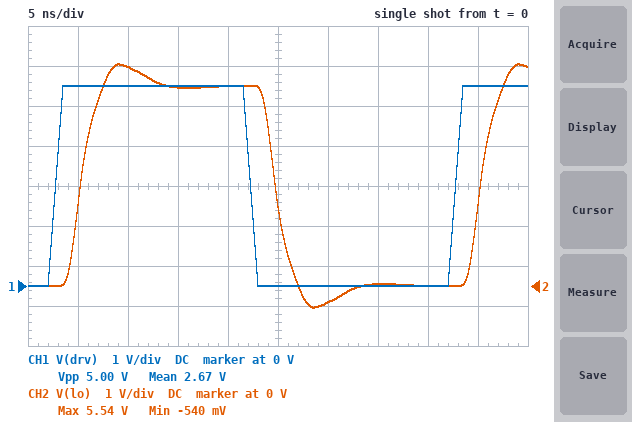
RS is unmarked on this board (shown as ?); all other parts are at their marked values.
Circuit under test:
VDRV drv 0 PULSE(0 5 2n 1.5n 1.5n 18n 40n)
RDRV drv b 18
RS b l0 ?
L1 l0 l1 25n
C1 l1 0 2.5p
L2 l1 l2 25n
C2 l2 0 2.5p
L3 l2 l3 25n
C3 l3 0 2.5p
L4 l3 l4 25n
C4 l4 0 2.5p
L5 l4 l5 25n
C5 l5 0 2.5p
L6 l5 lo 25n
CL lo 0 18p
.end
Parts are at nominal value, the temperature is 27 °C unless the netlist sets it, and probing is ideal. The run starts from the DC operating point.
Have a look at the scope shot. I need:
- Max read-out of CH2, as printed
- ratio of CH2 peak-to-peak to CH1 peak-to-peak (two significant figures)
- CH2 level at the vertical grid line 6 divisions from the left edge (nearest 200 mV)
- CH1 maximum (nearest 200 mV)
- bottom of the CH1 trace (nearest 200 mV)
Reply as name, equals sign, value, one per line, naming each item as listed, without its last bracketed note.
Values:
Max read-out of CH2, as printed = 5.54 V
ratio of CH2 peak-to-peak to CH1 peak-to-peak = 1.2
CH2 level at the vertical grid line 6 divisions from the left edge = -400 mV
CH1 maximum = 5.0 V
bottom of the CH1 trace = 0 V
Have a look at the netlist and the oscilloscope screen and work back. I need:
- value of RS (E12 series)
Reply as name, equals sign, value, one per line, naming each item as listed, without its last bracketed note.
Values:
value of RS = 56 Ω
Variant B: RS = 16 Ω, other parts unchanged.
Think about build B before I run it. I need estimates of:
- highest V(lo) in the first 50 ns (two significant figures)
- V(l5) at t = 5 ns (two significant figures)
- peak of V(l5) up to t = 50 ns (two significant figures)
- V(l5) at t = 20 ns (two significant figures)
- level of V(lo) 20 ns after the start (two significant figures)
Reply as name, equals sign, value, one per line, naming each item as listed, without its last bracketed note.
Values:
highest V(lo) in the first 50 ns = 7.5 V
V(l5) at t = 5 ns = 2.7 V
peak of V(l5) up to t = 50 ns = 7.1 V
V(l5) at t = 20 ns = 5.3 V
level of V(lo) 20 ns after the start = 5.4 V
